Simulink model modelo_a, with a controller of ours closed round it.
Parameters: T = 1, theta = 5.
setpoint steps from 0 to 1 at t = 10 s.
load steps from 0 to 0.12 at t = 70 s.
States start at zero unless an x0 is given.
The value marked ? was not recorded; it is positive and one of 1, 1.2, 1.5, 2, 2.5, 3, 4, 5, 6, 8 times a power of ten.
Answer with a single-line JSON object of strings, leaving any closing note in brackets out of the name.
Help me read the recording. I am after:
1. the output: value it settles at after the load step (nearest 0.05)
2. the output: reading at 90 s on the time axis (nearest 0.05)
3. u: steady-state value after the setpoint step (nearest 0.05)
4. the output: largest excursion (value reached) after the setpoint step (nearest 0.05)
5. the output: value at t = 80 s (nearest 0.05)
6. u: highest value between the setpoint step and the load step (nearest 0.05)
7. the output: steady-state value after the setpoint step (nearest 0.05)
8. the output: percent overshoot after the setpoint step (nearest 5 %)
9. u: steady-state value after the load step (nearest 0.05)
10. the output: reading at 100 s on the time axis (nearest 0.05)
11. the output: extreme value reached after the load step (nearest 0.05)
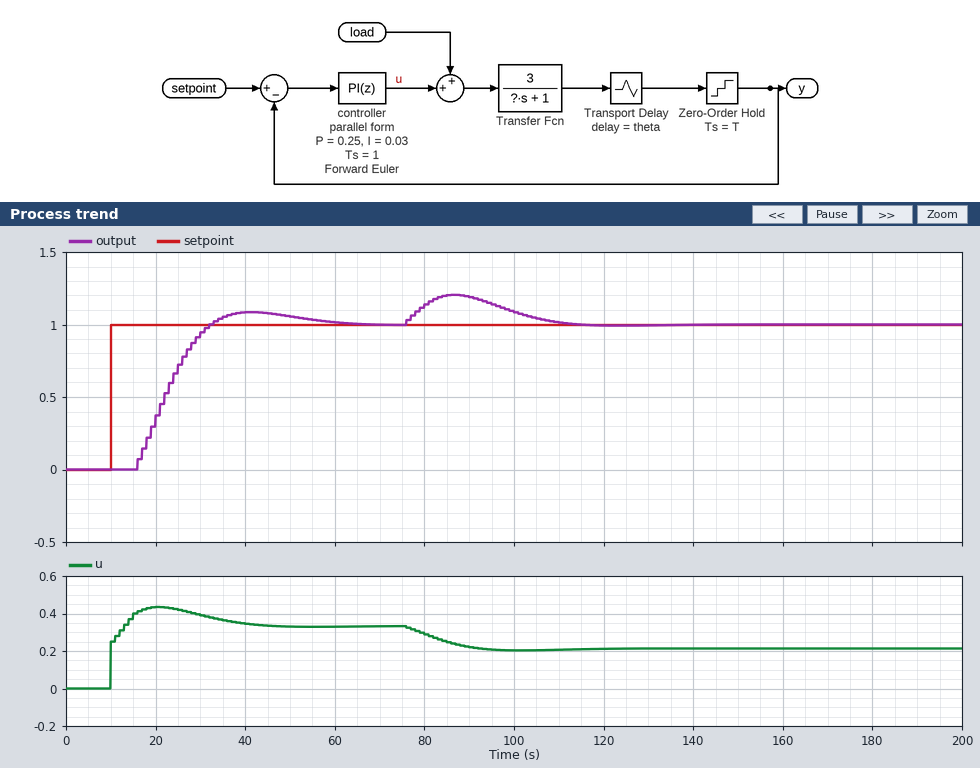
{"the output: value it settles at after the load step": "1.00", "the output: reading at 90 s on the time axis": "1.20", "u: steady-state value after the setpoint step": "0.35", "the output: largest excursion (value reached) after the setpoint step": "1.10", "the output: value at t = 80 s": "1.15", "u: highest value between the setpoint step and the load step": "0.45", "the output: steady-state value after the setpoint step": "1.00", "the output: percent overshoot after the setpoint step": "10 %", "u: steady-state value after the load step": "0.20", "the output: reading at 100 s on the time axis": "1.10", "the output: extreme value reached after the load step": "1.20"}
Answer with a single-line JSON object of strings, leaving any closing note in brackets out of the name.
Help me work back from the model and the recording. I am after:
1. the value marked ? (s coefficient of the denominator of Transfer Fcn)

{"the value marked ?": "10"}
